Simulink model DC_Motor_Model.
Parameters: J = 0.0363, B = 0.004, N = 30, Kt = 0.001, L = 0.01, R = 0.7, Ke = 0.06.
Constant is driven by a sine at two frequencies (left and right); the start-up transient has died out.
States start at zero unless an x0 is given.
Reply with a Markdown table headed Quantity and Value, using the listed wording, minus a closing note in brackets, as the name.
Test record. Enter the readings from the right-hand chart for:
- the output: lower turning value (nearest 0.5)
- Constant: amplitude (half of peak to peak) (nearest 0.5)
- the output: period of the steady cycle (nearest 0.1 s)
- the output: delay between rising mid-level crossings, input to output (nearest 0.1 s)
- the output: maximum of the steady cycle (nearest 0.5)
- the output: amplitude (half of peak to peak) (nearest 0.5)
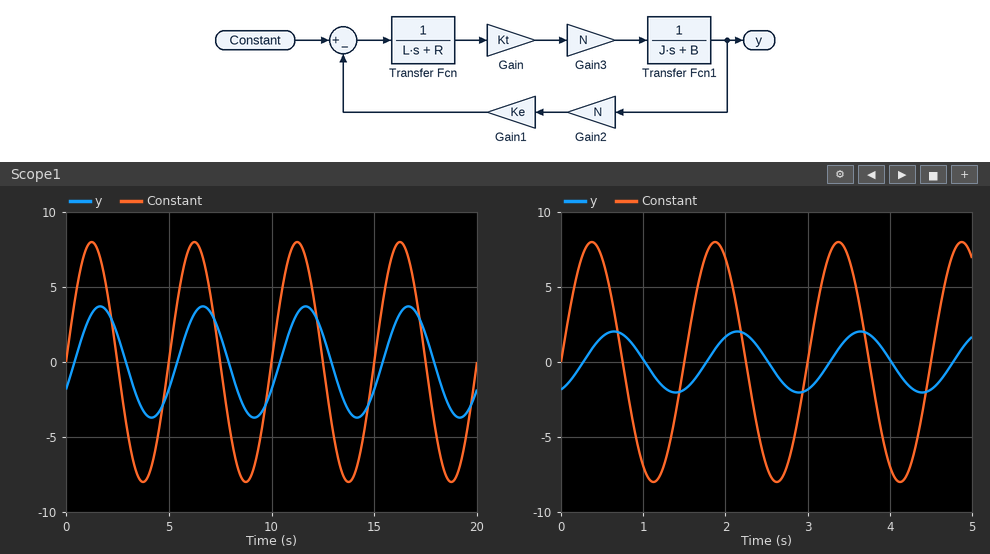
| Quantity | Value |
|---|---|
| the output: lower turning value | -2.0 |
| Constant: amplitude (half of peak to peak) | 8.0 |
| the output: period of the steady cycle | 1.5 s |
| the output: delay between rising mid-level crossings, input to output | 0.3 s |
| the output: maximum of the steady cycle | 2.0 |
| the output: amplitude (half of peak to peak) | 2.0 |
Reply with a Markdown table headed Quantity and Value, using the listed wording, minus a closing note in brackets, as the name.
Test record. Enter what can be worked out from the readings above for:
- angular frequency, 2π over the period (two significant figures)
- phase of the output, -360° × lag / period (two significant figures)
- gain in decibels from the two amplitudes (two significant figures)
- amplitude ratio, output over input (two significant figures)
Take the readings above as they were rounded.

| Quantity | Value |
|---|---|
| angular frequency, 2π over the period | 4.2 rad/s |
| phase of the output, -360° × lag / period | -72° |
| gain in decibels from the two amplitudes | -12 dB |
| amplitude ratio, output over input | 0.25 |
